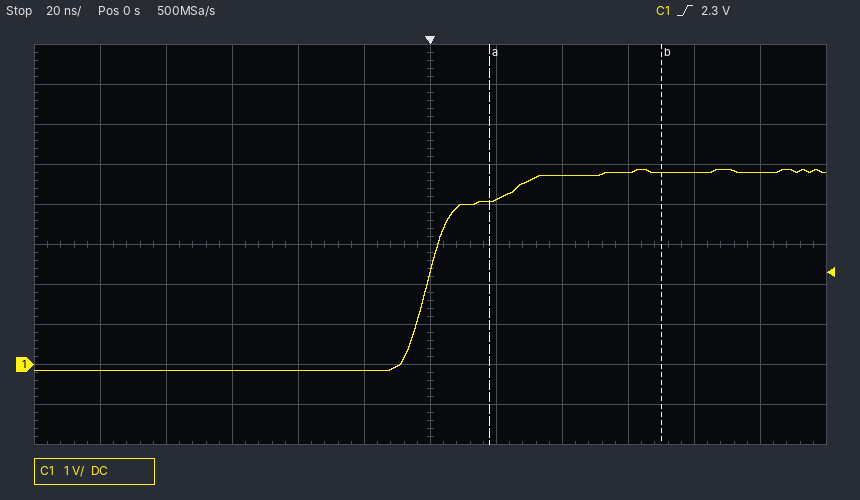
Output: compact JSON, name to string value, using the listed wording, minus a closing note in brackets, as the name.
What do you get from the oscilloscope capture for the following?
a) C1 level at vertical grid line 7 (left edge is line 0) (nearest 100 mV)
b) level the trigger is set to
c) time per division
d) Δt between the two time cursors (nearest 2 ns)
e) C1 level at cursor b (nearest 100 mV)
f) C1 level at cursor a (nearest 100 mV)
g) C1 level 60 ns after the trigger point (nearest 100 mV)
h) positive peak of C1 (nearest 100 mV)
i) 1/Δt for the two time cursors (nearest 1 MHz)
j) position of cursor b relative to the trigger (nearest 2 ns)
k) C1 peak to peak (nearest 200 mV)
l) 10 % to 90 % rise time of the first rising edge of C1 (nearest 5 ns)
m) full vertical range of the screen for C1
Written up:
{"C1 level at vertical grid line 7 (left edge is line 0)": "4.1 V", "level the trigger is set to": "2.3 V", "time per division": "20 ns", "Δt between the two time cursors": "52 ns", "C1 level at cursor b": "4.8 V", "C1 level at cursor a": "4.1 V", "C1 level 60 ns after the trigger point": "4.8 V", "positive peak of C1": "4.9 V", "1/Δt for the two time cursors": "19 MHz", "position of cursor b relative to the trigger": "+70 ns", "C1 peak to peak": "5.0 V", "10 % to 90 % rise time of the first rising edge of C1": "30 ns", "full vertical range of the screen for C1": "10 V"}
